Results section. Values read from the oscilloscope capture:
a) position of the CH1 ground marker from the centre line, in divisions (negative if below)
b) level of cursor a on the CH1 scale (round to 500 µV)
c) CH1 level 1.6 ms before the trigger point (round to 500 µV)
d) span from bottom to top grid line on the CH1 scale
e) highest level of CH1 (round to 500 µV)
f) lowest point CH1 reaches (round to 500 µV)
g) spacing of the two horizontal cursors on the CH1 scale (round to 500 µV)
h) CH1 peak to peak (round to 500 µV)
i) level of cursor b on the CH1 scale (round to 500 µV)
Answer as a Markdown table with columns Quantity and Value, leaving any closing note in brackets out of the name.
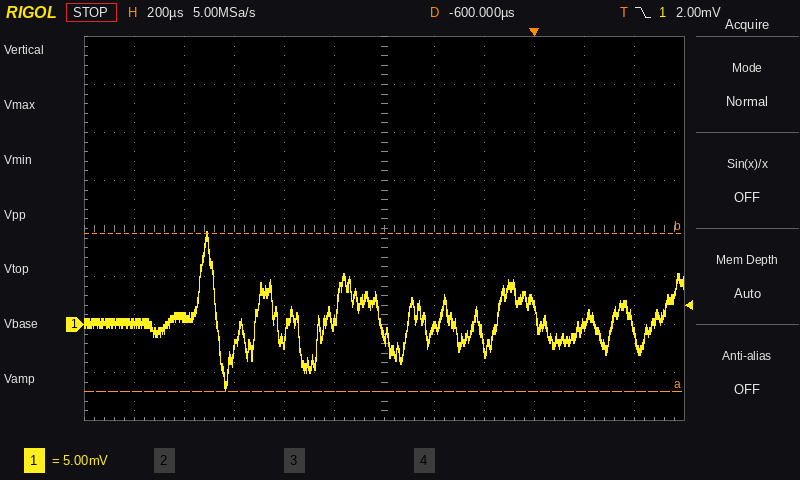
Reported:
| Quantity | Value |
|---|---|
| position of the CH1 ground marker from the centre line, in divisions | -2.0 div |
| level of cursor a on the CH1 scale | -7.0 mV |
| CH1 level 1.6 ms before the trigger point | 0.0 mV |
| span from bottom to top grid line on the CH1 scale | 40 mV |
| highest level of CH1 | 9.5 mV |
| lowest point CH1 reaches | -7.0 mV |
| spacing of the two horizontal cursors on the CH1 scale | 16.5 mV |
| CH1 peak to peak | 16.5 mV |
| level of cursor b on the CH1 scale | 9.5 mV |
